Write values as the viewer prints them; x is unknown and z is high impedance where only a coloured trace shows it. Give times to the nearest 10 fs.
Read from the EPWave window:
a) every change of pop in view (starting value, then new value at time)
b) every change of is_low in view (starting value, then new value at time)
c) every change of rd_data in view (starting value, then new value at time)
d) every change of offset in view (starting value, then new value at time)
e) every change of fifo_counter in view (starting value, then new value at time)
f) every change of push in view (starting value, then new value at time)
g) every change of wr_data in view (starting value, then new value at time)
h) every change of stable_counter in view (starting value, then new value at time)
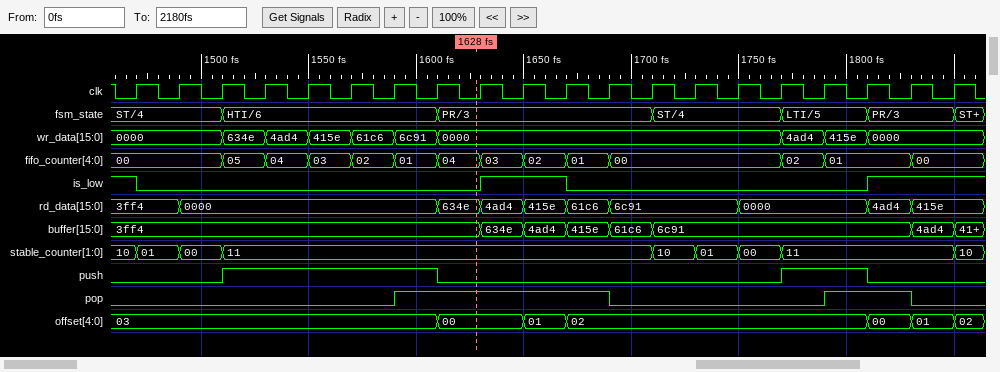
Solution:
0, 1 at 1590 fs, 0 at 1690 fs, 1 at 1790 fs, 0 at 1830 fs
1, 0 at 1470 fs, 1 at 1630 fs, 0 at 1670 fs, 1 at 1810 fs
3ff4, 0000 at 1490 fs, 634e at 1610 fs, 4ad4 at 1630 fs, 415e at 1650 fs, 61c6 at 1670 fs, 6c91 at 1690 fs, 0000 at 1750 fs, 4ad4 at 1810 fs, 415e at 1830 fs
03, 00 at 1610 fs, 01 at 1650 fs, 02 at 1670 fs, 00 at 1810 fs, 01 at 1830 fs, 02 at 1850 fs
00, 05 at 1510 fs, 04 at 1530 fs, 03 at 1550 fs, 02 at 1570 fs, 01 at 1590 fs, 04 at 1610 fs, 03 at 1630 fs, 02 at 1650 fs, 01 at 1670 fs, 00 at 1690 fs, 02 at 1770 fs, 01 at 1790 fs, 00 at 1830 fs
0, 1 at 1510 fs, 0 at 1610 fs, 1 at 1770 fs, 0 at 1810 fs
0000, 634e at 1510 fs, 4ad4 at 1530 fs, 415e at 1550 fs, 61c6 at 1570 fs, 6c91 at 1590 fs, 0000 at 1610 fs, 4ad4 at 1770 fs, 415e at 1790 fs, 0000 at 1810 fs
10, 01 at 1470 fs, 00 at 1490 fs, 11 at 1510 fs, 10 at 1710 fs, 01 at 1730 fs, 00 at 1750 fs, 11 at 1770 fs, 10 at 1850 fs
